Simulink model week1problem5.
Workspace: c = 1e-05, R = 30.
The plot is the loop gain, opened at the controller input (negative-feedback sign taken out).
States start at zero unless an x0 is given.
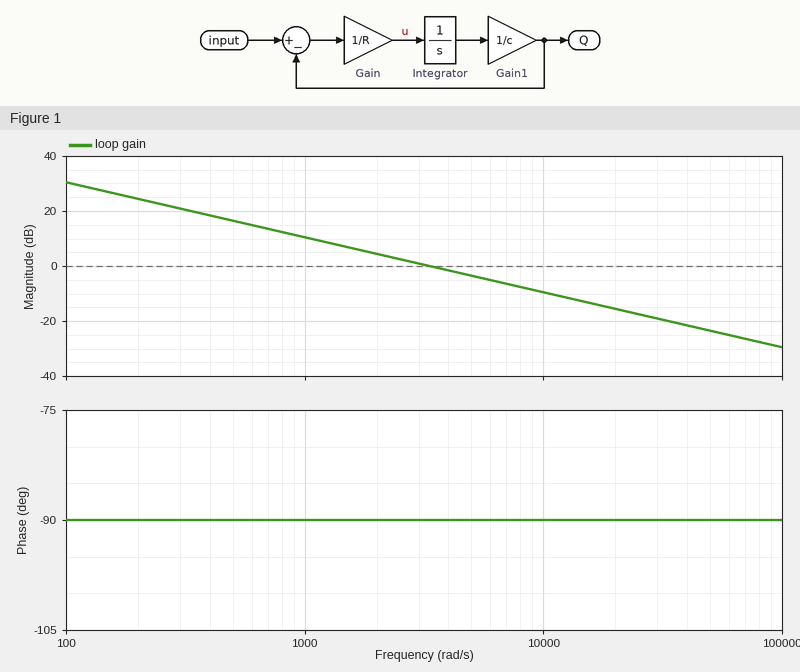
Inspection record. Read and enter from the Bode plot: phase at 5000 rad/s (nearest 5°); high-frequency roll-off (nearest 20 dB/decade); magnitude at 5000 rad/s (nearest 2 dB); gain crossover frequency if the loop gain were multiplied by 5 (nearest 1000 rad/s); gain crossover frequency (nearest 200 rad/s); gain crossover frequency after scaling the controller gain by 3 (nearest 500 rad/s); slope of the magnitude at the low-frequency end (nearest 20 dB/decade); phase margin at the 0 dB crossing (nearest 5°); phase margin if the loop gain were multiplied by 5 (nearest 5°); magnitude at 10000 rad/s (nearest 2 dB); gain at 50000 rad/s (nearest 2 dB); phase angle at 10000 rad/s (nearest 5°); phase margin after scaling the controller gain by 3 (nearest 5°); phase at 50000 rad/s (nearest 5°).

-90°
-20 dB/decade
-4 dB
17000 rad/s
3400 rad/s
10000 rad/s
-20 dB/decade
90°
90°
-10 dB
-24 dB
-90°
90°
-90°
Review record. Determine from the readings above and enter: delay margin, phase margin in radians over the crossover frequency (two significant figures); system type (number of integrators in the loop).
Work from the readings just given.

0.00046 s
1
